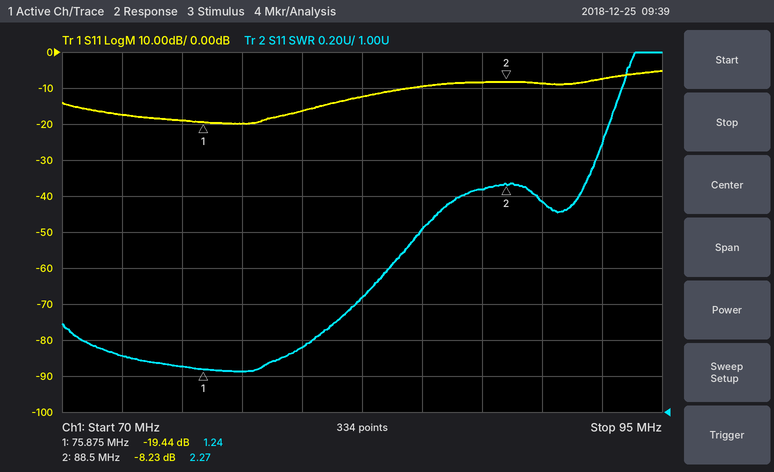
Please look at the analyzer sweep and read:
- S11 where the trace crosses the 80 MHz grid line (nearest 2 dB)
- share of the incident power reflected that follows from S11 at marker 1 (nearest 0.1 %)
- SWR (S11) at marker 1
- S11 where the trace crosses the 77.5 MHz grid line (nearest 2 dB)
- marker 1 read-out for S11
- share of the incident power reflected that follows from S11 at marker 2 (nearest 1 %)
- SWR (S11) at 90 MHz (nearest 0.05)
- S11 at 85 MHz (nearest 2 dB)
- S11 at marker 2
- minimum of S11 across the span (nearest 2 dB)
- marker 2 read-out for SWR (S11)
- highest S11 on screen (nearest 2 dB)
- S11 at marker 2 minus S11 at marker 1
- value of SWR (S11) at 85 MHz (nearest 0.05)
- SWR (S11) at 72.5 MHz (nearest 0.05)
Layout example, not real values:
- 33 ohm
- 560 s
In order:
- -16 dB
- 1.1 %
- 1.24
- -20 dB
- -19.44 dB
- 15 %
- 2.15
- -10 dB
- -8.23 dB
- -20 dB
- 2.27
- -6 dB
- 11.21 dB
- 2.00
- 1.30
